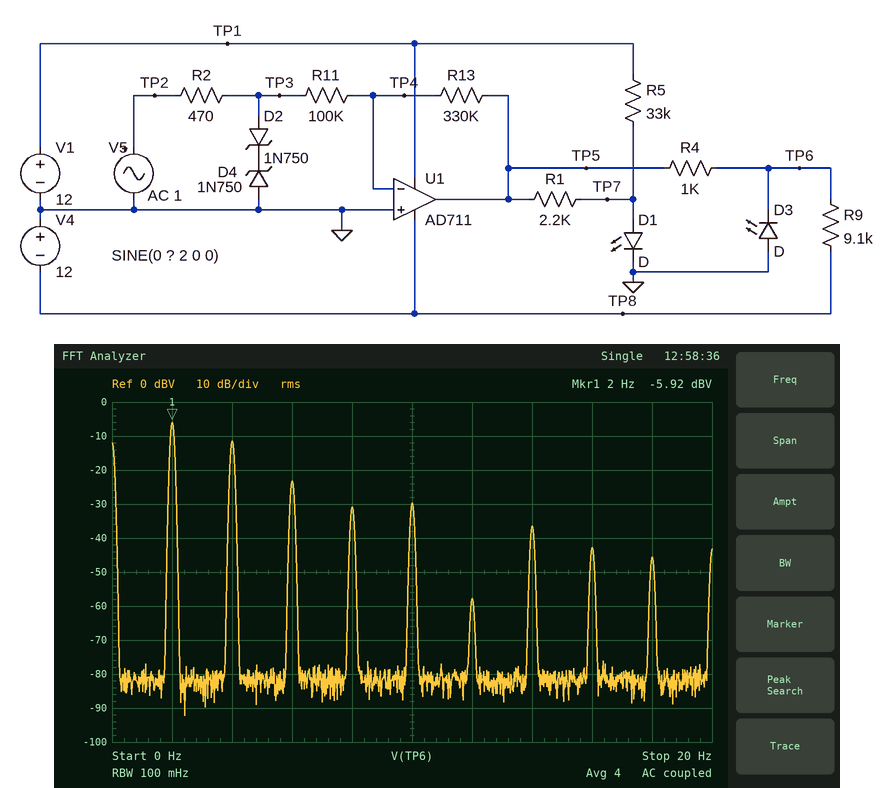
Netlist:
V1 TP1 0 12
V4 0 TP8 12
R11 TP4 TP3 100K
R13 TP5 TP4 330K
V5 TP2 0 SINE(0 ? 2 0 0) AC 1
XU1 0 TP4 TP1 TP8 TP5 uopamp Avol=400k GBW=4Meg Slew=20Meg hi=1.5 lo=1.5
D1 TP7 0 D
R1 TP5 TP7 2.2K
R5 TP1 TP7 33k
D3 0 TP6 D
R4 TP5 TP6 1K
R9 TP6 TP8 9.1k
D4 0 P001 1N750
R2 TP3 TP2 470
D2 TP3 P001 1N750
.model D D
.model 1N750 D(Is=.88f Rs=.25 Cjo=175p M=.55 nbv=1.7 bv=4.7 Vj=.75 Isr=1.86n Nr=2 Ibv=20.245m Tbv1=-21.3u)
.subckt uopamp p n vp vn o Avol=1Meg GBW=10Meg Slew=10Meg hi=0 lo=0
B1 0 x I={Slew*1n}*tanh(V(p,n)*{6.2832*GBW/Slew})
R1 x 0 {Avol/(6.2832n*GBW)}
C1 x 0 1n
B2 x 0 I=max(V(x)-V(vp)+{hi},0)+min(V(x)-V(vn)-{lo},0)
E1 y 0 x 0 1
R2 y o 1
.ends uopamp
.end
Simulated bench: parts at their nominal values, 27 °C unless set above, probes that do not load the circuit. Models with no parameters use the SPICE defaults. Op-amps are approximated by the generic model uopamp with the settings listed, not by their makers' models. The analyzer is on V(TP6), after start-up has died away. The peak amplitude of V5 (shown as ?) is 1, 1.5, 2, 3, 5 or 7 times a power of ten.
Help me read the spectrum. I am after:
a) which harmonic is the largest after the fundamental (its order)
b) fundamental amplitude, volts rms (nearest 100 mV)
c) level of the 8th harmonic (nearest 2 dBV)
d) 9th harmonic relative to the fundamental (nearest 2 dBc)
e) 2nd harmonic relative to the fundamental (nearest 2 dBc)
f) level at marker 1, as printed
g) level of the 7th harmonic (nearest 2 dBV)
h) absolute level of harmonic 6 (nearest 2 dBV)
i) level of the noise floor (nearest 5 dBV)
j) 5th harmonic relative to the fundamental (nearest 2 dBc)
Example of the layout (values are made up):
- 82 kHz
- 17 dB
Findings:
- 2
- 500 mV
- -42 dBV
- -40 dBc
- -6 dBc
- -5.92 dBV
- -36 dBV
- -58 dBV
- -80 dBV
- -24 dBc
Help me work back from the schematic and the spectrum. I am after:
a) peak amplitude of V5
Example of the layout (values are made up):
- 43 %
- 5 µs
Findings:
- 700 mV
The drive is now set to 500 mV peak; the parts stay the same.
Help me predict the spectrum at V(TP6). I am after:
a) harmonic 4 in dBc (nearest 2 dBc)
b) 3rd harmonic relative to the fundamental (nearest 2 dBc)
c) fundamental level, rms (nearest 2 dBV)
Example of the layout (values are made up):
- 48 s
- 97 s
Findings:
- -38 dBc
- -14 dBc
- -10 dBV
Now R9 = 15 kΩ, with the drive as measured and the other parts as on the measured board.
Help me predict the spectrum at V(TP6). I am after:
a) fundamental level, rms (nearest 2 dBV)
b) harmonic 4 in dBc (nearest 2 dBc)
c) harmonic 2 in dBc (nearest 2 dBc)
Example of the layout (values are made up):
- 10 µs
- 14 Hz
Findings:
- -2 dBV
- -22 dBc
- -8 dBc
